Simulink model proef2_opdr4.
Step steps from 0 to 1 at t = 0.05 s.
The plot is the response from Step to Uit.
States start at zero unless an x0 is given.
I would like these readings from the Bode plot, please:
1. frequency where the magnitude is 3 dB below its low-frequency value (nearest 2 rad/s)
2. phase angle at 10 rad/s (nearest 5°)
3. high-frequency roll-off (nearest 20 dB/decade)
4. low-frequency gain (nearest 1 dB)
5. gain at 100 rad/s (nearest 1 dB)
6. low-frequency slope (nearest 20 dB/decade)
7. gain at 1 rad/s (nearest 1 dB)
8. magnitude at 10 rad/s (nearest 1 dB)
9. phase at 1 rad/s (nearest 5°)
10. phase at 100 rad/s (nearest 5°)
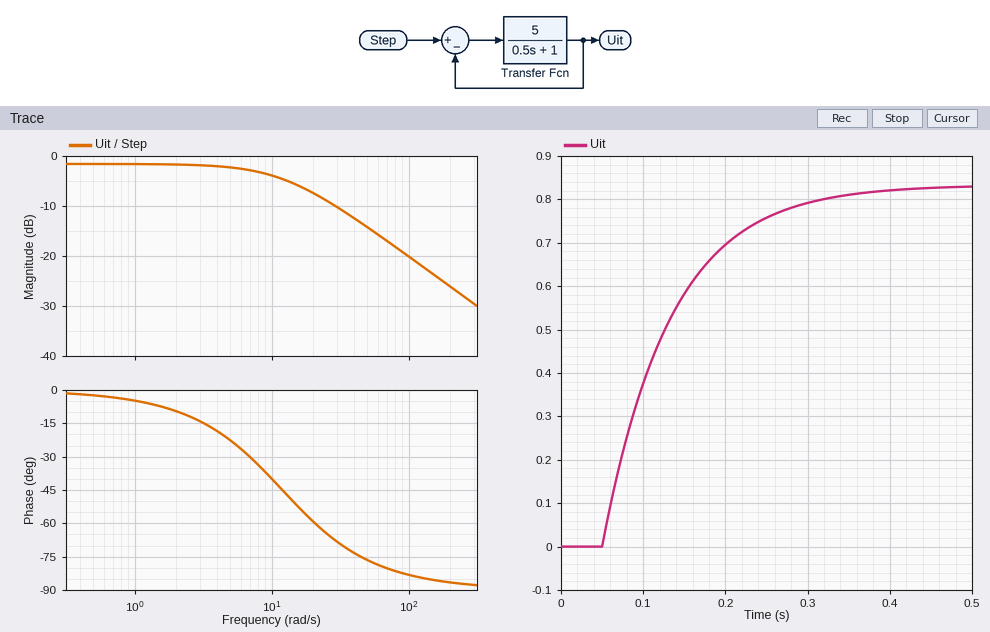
12 rad/s
-40°
-20 dB/decade
-2 dB
-20 dB
0 dB/decade
-2 dB
-4 dB
-5°
-85°
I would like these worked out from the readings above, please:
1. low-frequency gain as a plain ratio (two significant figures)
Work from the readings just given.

0.79
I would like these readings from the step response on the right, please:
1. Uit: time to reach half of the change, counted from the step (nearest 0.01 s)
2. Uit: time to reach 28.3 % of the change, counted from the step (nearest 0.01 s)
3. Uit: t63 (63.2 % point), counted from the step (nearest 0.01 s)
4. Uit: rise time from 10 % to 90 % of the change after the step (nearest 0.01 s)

0.06 s
0.03 s
0.08 s
0.18 s
